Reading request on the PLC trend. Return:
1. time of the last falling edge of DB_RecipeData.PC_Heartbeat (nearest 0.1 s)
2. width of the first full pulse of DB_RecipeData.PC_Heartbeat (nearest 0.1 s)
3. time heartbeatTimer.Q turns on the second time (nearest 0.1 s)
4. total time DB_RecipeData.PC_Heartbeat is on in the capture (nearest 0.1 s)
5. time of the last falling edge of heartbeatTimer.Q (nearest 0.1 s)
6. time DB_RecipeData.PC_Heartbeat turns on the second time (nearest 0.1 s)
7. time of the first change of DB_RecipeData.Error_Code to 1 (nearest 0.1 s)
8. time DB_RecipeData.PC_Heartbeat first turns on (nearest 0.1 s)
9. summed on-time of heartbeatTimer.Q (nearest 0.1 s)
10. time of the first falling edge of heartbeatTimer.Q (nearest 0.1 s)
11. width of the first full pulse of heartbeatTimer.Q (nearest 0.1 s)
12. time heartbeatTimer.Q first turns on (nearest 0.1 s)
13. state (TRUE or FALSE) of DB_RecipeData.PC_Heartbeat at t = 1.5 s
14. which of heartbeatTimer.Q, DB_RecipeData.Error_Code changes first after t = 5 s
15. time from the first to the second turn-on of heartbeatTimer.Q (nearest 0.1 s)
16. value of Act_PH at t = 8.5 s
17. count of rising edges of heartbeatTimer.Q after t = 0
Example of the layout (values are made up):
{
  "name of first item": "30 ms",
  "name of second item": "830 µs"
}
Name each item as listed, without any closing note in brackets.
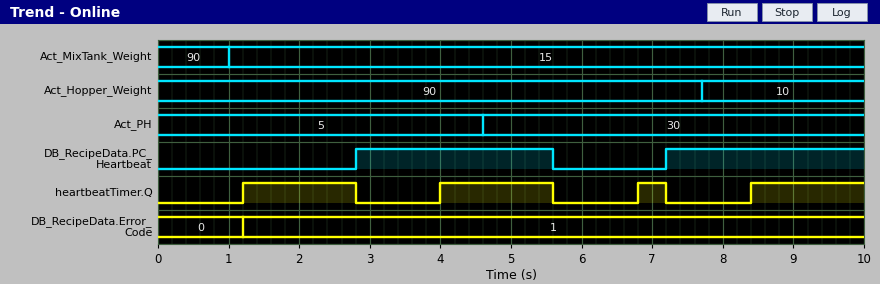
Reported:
{
  "time of the last falling edge of DB_RecipeData.PC_Heartbeat": "5.6 s",
  "width of the first full pulse of DB_RecipeData.PC_Heartbeat": "2.8 s",
  "time heartbeatTimer.Q turns on the second time": "4.0 s",
  "total time DB_RecipeData.PC_Heartbeat is on in the capture": "5.6 s",
  "time of the last falling edge of heartbeatTimer.Q": "7.2 s",
  "time DB_RecipeData.PC_Heartbeat turns on the second time": "7.2 s",
  "time of the first change of DB_RecipeData.Error_Code to 1": "1.2 s",
  "time DB_RecipeData.PC_Heartbeat first turns on": "2.8 s",
  "summed on-time of heartbeatTimer.Q": "5.2 s",
  "time of the first falling edge of heartbeatTimer.Q": "2.8 s",
  "width of the first full pulse of heartbeatTimer.Q": "1.6 s",
  "time heartbeatTimer.Q first turns on": "1.2 s",
  "state (TRUE or FALSE) of DB_RecipeData.PC_Heartbeat at t = 1.5 s": "FALSE",
  "which of heartbeatTimer.Q, DB_RecipeData.Error_Code changes first after t = 5 s": "heartbeatTimer.Q",
  "time from the first to the second turn-on of heartbeatTimer.Q": "2.8 s",
  "value of Act_PH at t = 8.5 s": "30",
  "count of rising edges of heartbeatTimer.Q after t = 0": "4"
}
